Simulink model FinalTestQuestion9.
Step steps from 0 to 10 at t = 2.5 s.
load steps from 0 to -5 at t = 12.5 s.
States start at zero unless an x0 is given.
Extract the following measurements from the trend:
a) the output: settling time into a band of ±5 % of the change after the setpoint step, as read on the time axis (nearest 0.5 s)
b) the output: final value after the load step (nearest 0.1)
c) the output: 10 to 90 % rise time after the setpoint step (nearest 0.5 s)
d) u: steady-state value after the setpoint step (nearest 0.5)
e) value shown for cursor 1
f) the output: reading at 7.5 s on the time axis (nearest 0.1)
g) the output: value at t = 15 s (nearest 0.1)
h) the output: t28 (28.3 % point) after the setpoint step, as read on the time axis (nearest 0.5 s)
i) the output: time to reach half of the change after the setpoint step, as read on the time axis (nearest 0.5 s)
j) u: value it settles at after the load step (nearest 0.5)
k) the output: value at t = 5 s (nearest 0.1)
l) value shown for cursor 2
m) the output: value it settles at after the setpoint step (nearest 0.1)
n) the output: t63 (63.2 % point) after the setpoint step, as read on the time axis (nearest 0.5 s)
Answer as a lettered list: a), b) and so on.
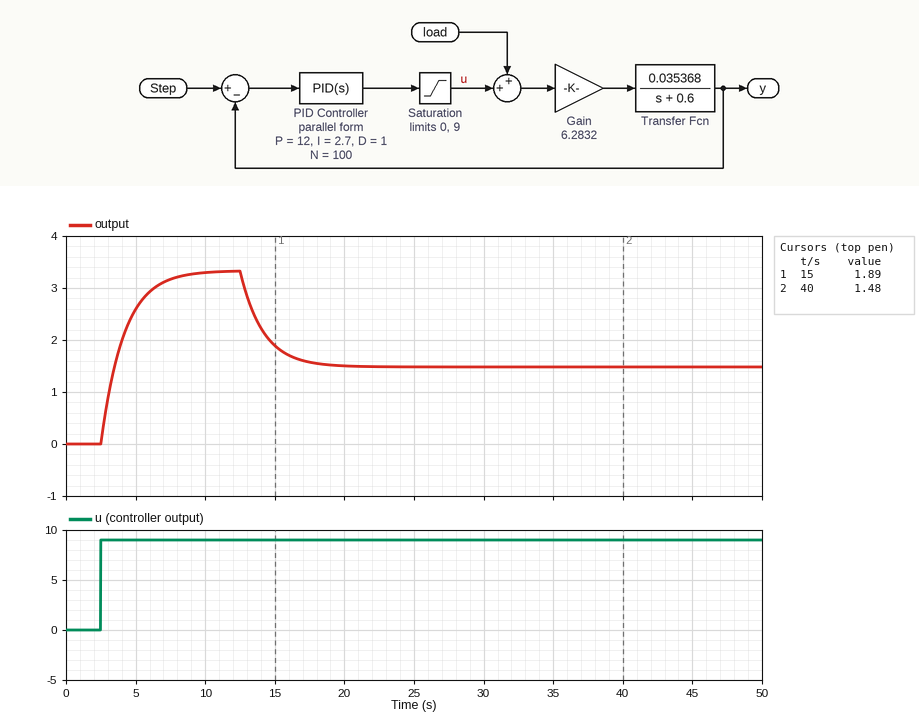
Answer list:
a) 7.5 s
b) 1.5
c) 3.5 s
d) 9.0
e) 1.89
f) 3.2
g) 1.9
h) 3.0 s
i) 3.5 s
j) 9.0
k) 2.6
l) 1.48
m) 3.3
n) 4.0 s
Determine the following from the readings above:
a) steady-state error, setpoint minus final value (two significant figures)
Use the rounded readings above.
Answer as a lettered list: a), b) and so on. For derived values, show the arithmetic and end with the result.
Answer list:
a) 10 - 3.3 = 6.7
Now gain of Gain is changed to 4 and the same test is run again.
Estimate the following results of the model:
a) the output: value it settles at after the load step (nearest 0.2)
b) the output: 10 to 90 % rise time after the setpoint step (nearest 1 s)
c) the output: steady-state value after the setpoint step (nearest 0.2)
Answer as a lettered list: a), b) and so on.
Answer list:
a) 1.0
b) 4 s
c) 2.2
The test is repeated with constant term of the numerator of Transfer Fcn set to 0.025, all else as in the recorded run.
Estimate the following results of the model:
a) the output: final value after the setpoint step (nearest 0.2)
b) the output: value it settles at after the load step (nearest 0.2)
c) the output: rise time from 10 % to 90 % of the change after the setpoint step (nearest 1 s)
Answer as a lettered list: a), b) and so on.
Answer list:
a) 2.4
b) 1.0
c) 4 s
